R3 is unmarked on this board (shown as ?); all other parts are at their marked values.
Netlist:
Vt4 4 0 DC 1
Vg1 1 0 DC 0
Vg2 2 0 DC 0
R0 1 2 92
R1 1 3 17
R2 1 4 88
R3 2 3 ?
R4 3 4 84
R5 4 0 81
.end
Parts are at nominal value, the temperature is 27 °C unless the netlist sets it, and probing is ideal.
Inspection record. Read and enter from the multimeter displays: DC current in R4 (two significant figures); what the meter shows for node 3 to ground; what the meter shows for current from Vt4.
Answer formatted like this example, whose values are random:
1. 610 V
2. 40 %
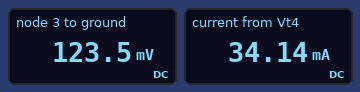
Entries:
1. 10 mA
2. 123.5 mV
3. 34.14 mA
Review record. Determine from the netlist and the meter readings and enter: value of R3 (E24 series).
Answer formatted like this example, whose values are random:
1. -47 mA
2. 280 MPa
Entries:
1. 39 Ω
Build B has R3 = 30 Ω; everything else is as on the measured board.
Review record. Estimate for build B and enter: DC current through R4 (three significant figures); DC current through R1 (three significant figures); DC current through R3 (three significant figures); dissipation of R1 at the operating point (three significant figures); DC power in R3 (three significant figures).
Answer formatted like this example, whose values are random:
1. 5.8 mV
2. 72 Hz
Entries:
1. 10.5 mA
2. 6.73 mA
3. 3.81 mA
4. 770 µW
5. 436 µW
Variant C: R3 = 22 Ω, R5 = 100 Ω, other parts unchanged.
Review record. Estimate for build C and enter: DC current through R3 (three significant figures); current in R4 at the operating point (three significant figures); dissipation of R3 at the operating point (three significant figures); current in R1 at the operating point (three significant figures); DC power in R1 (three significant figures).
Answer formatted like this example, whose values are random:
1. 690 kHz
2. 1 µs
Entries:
1. 4.66 mA
2. 10.7 mA
3. 477 µW
4. 6.03 mA
5. 618 µW
